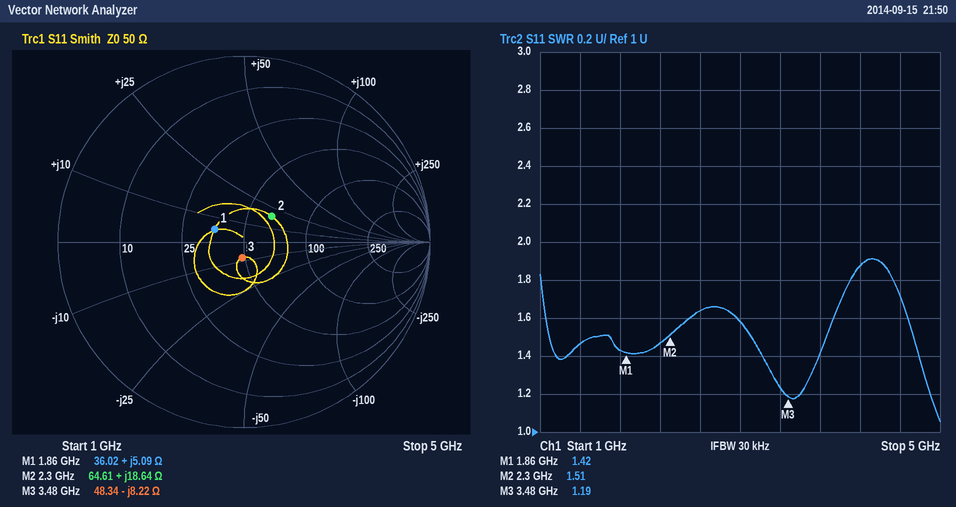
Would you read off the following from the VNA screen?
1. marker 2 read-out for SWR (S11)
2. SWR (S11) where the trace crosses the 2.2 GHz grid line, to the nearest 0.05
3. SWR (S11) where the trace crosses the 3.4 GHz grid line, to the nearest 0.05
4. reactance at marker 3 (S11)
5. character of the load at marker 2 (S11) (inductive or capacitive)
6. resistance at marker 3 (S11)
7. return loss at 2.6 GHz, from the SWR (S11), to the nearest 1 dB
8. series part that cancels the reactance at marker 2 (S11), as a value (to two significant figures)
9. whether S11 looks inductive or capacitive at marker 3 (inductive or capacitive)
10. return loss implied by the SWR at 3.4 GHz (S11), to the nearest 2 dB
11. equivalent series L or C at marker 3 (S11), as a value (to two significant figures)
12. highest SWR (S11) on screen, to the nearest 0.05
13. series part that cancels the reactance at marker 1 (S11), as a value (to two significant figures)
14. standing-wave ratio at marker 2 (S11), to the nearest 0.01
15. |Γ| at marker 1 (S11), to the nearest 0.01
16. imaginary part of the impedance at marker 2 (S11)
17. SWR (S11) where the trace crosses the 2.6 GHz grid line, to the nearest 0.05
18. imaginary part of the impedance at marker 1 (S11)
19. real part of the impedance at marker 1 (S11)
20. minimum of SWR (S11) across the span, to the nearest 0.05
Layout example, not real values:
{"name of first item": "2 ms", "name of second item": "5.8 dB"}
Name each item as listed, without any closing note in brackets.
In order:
{"marker 2 read-out for SWR": "1.51", "SWR (S11) where the trace crosses the 2.2 GHz grid line, to the nearest 0.05": "1.45", "SWR (S11) where the trace crosses the 3.4 GHz grid line, to the nearest 0.05": "1.25", "reactance at marker 3": "-8.22 Ω", "character of the load at marker 2 (S11)": "inductive", "resistance at marker 3": "48.34 Ω", "return loss at 2.6 GHz, from the SWR (S11), to the nearest 1 dB": "12 dB", "series part that cancels the reactance at marker 2 (S11), as a value": "3.7 pF", "whether S11 looks inductive or capacitive at marker 3": "capacitive", "return loss implied by the SWR at 3.4 GHz (S11), to the nearest 2 dB": "20 dB", "equivalent series L or C at marker 3 (S11), as a value": "5.6 pF", "highest SWR (S11) on screen, to the nearest 0.05": "1.90", "series part that cancels the reactance at marker 1 (S11), as a value": "17 pF", "standing-wave ratio at marker 2 (S11), to the nearest 0.01": "1.51", "|Γ| at marker 1 (S11), to the nearest 0.01": "0.17", "imaginary part of the impedance at marker 2": "+18.64 Ω", "SWR (S11) where the trace crosses the 2.6 GHz grid line, to the nearest 0.05": "1.65", "imaginary part of the impedance at marker 1": "+5.09 Ω", "real part of the impedance at marker 1": "36.02 Ω", "minimum of SWR (S11) across the span, to the nearest 0.05": "1.05"}
